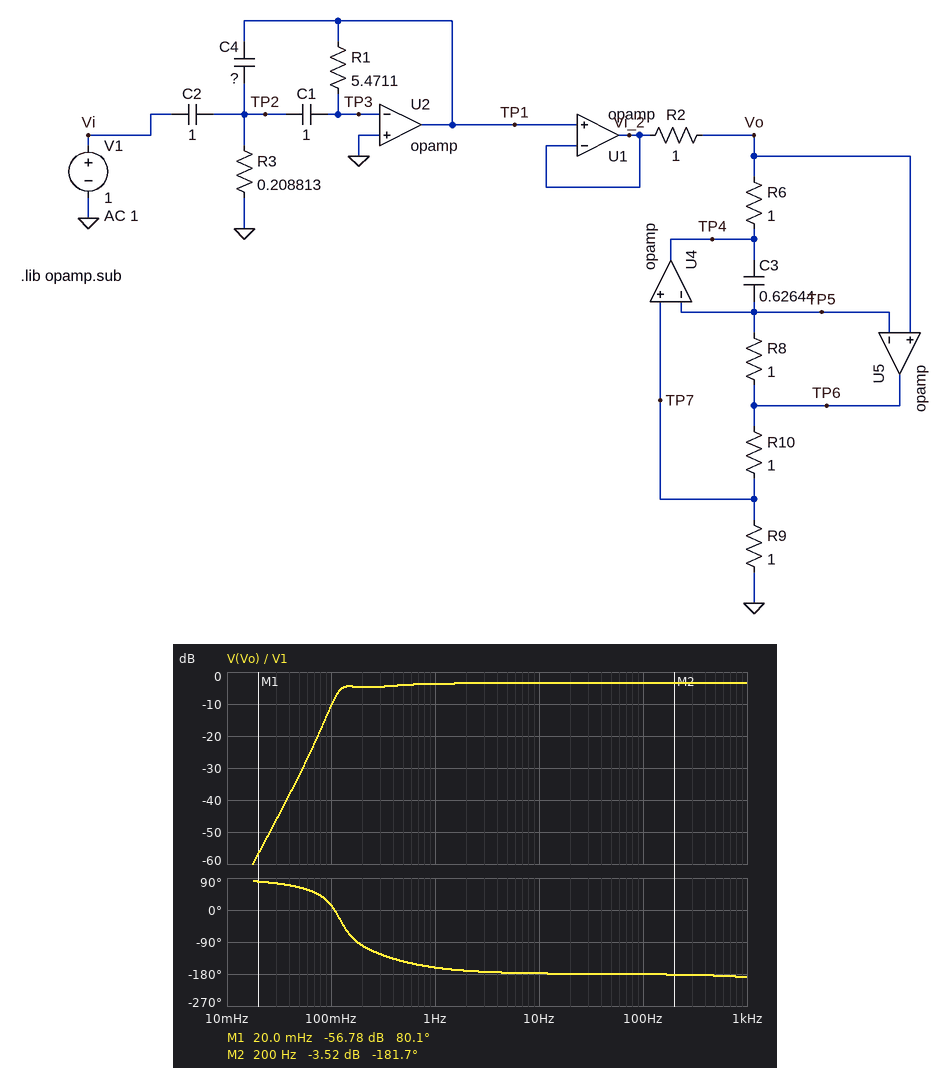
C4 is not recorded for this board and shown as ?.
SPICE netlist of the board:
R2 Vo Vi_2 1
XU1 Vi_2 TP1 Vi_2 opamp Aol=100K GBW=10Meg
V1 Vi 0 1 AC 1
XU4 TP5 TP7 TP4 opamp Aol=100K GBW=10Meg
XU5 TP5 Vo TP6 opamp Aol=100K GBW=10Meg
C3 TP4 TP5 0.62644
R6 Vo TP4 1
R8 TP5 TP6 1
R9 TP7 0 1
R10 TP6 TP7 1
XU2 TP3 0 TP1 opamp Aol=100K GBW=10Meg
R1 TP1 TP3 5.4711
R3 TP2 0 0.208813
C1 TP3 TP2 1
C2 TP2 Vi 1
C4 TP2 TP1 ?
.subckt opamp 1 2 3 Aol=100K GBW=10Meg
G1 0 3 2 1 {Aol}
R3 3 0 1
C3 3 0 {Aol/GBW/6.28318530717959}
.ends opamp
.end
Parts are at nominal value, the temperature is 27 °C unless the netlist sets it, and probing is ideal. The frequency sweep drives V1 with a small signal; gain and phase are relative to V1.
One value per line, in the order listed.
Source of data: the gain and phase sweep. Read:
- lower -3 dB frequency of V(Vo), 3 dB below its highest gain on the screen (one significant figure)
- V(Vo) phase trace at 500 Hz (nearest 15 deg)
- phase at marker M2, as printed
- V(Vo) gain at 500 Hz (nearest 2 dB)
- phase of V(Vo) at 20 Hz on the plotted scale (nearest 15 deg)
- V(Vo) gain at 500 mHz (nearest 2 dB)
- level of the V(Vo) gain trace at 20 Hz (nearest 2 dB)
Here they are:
100 mHz
-180 deg
-181.7 deg
-4 dB
-180 deg
-4 dB
-4 dB
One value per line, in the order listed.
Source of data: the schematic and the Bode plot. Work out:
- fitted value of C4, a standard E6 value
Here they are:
1.5 F
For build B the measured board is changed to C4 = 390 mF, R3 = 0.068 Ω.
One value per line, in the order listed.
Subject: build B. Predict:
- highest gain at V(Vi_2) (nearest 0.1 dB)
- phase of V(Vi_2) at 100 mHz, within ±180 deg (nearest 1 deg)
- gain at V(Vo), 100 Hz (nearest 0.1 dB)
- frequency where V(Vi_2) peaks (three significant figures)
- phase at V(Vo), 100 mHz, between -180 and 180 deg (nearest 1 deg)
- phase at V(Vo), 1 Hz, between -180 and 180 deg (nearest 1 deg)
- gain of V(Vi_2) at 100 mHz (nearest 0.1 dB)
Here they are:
15.8 dB
-6 deg
8.2 dB
438 mHz
62 deg
-154 deg
-16.2 dB
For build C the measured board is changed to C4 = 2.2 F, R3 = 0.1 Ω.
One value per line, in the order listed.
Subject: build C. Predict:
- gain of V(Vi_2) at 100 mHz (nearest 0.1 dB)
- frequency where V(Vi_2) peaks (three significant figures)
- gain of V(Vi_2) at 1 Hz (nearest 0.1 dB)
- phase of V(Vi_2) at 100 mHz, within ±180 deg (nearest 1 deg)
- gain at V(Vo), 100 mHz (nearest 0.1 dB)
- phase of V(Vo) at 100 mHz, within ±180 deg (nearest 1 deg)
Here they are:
-8.7 dB
151 mHz
-6.7 dB
-27 deg
-17.4 dB
42 deg
